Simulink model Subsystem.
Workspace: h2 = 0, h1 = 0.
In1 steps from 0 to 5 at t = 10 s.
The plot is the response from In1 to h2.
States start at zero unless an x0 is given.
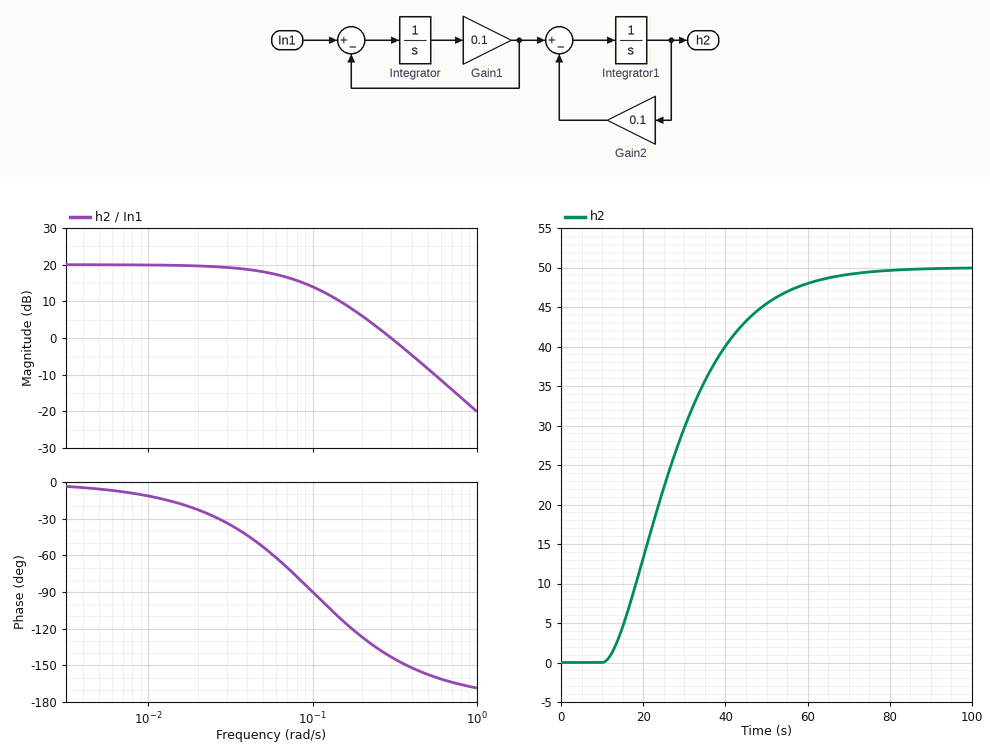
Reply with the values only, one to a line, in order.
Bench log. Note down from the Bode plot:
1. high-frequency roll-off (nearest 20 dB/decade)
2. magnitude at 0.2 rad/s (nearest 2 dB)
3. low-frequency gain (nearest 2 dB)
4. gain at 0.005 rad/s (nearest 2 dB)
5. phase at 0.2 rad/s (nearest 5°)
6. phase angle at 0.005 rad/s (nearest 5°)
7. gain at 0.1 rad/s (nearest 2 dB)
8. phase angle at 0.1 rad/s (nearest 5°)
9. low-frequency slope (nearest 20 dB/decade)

-40 dB/decade
6 dB
20 dB
20 dB
-125°
-5°
14 dB
-90°
0 dB/decade
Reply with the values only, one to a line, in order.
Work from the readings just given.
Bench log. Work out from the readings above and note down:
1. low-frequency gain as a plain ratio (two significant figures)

10
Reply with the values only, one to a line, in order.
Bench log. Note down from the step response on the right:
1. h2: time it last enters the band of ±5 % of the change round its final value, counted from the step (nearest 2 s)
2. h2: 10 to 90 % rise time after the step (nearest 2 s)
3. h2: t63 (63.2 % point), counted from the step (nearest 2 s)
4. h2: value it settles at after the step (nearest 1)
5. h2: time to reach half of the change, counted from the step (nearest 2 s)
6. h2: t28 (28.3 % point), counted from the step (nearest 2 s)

48 s
34 s
22 s
50
16 s
10 s
